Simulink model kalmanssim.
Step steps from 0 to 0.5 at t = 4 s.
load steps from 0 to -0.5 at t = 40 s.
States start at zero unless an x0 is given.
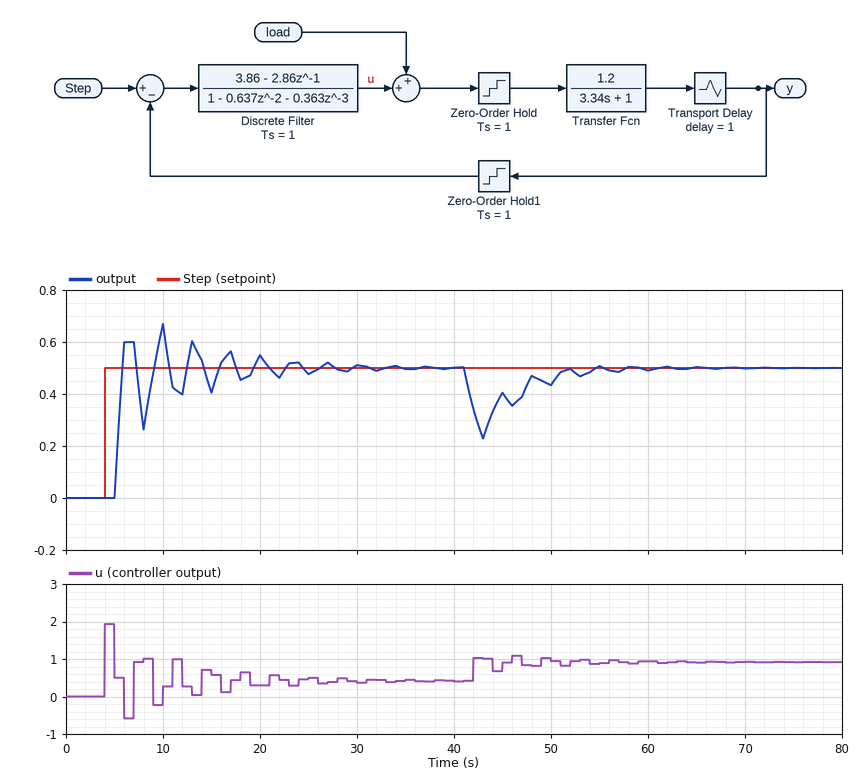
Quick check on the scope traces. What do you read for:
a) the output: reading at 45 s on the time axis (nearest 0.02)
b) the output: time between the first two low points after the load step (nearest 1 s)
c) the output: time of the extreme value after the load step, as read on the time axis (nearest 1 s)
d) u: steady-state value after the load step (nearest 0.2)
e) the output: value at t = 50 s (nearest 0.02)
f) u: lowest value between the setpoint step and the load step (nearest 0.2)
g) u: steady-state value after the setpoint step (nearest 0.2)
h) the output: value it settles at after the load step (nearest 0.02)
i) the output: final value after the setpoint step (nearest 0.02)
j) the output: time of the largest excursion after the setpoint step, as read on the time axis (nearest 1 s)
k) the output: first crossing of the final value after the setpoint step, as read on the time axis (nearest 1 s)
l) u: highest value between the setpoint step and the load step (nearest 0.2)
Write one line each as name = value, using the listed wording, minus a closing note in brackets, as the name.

the output: reading at 45 s on the time axis = 0.40
the output: time between the first two low points after the load step = 3 s
the output: time of the extreme value after the load step, as read on the time axis = 43 s
u: steady-state value after the load step = 1.0
the output: value at t = 50 s = 0.44
u: lowest value between the setpoint step and the load step = -0.6
u: steady-state value after the setpoint step = 0.4
the output: value it settles at after the load step = 0.50
the output: final value after the setpoint step = 0.50
the output: time of the largest excursion after the setpoint step, as read on the time axis = 10 s
the output: first crossing of the final value after the setpoint step, as read on the time axis = 6 s
u: highest value between the setpoint step and the load step = 2.0
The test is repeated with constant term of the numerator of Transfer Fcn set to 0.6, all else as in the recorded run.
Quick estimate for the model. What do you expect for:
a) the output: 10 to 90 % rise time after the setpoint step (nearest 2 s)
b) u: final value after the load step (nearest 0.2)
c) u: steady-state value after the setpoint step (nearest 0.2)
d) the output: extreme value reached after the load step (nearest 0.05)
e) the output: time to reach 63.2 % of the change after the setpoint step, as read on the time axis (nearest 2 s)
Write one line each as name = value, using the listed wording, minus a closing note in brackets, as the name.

the output: 10 to 90 % rise time after the setpoint step = 6 s
u: final value after the load step = 1.4
u: steady-state value after the setpoint step = 0.8
the output: extreme value reached after the load step = 0.35
the output: time to reach 63.2 % of the change after the setpoint step, as read on the time axis = 8 s
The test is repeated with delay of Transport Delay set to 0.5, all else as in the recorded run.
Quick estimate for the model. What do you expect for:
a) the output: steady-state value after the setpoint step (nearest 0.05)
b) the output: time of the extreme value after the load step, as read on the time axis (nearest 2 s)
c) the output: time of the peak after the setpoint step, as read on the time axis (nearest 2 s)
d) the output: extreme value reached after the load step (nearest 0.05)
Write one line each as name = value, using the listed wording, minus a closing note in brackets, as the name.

the output: steady-state value after the setpoint step = 0.50
the output: time of the extreme value after the load step, as read on the time axis = 42 s
the output: time of the peak after the setpoint step, as read on the time axis = 6 s
the output: extreme value reached after the load step = 0.35
